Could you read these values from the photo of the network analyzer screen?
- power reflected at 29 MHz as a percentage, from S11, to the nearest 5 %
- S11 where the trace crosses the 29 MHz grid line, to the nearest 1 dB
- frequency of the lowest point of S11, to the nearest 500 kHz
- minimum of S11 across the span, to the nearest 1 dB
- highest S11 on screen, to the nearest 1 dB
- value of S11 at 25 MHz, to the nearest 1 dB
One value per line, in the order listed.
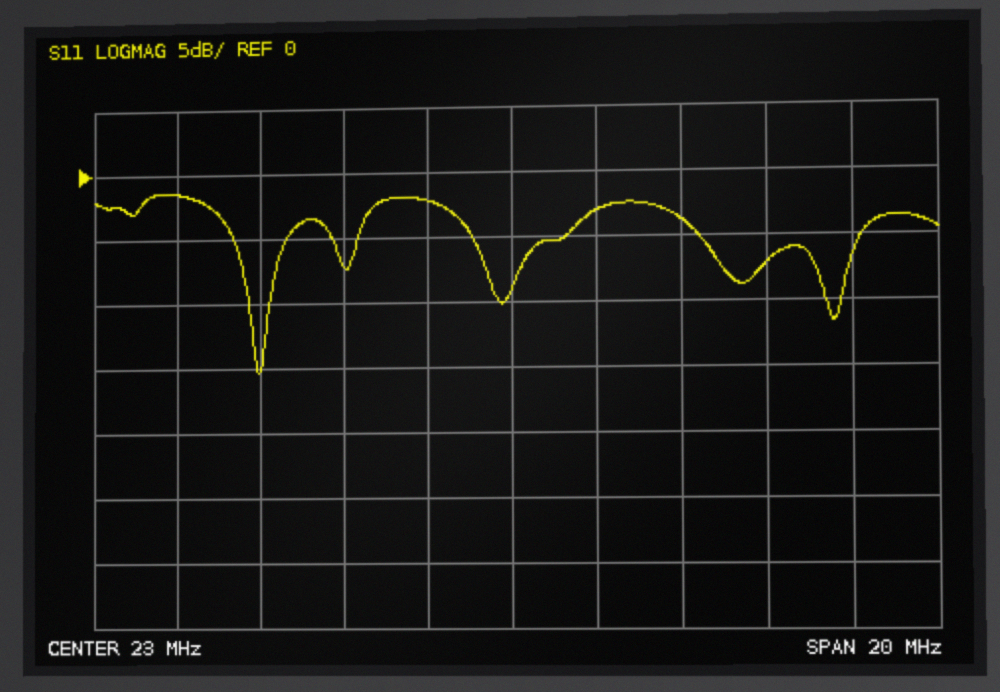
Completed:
20 %
-7 dB
17.0 MHz
-15 dB
-1 dB
-3 dB
